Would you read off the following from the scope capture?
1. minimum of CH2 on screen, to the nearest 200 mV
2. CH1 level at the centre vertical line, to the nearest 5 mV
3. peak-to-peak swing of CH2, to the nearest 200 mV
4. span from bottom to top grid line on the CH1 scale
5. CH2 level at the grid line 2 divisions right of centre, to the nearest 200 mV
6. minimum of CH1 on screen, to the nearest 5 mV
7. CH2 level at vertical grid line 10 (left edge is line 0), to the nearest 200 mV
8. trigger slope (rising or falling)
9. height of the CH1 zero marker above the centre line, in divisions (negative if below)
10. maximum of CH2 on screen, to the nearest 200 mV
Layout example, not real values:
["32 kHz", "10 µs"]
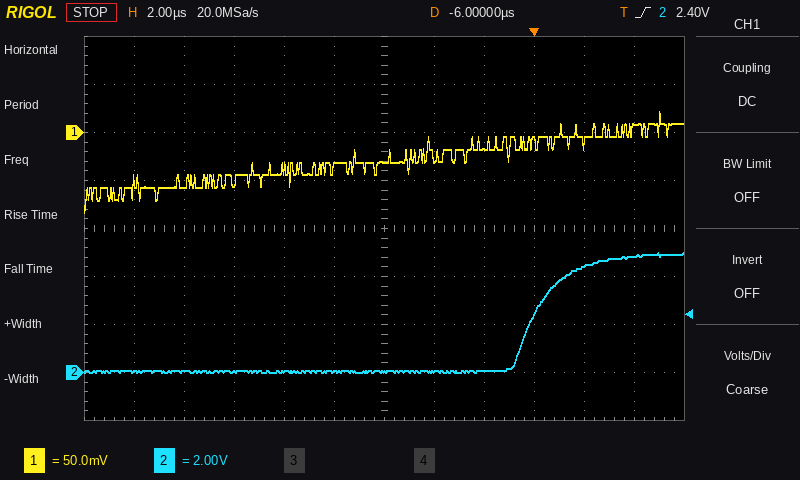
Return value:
["0.0 V", "-30 mV", "5.0 V", "400 mV", "0.0 V", "-85 mV", "4.4 V", "rising", "+2.0 div", "5.0 V"]
